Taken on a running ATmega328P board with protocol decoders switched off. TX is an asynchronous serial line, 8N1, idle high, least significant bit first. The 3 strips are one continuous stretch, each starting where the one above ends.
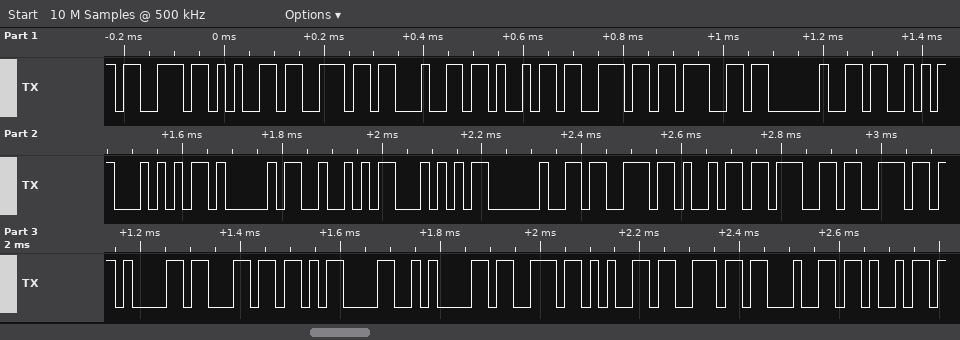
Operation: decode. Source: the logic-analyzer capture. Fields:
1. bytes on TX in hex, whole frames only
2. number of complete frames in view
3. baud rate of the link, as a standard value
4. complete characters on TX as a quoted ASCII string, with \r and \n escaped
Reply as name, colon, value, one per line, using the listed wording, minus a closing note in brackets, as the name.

bytes on TX in hex, whole frames only: 73 65 6E 64 69 6E 67 20 53 54 41 52 54 20 73 69 67 6E 61 6C 0D 0A 73 65 6E 64 69
number of complete frames in view: 27
baud rate of the link, as a standard value: 57600 baud
complete characters on TX as a quoted ASCII string, with \r and \n escaped: "sending START signal\r\nsendi"
